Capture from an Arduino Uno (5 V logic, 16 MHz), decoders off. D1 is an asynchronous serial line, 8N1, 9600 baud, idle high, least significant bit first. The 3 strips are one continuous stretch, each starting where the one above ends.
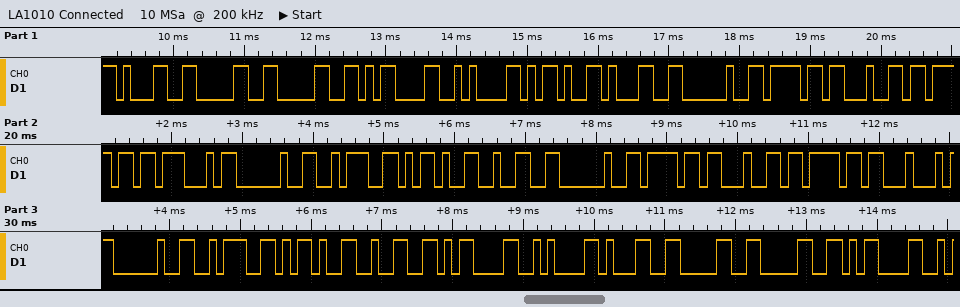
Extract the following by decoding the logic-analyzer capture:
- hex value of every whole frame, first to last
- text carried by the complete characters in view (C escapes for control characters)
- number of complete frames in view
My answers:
0x31 0x30 0x30 0x0D 0x0A 0x2D 0x31 0x20 0x6F 0x64 0x6F 0x47 0x20 0x3A 0x2D 0x32 0x20 0x6F 0x64 0x6F 0x44 0x20 0x3A 0x2D 0x32 0x0D 0x0A 0x31 0x30 0x30 0x0D
"100\r\n-1 odoG :-2 odoD :-2\r\n100\r"
31
